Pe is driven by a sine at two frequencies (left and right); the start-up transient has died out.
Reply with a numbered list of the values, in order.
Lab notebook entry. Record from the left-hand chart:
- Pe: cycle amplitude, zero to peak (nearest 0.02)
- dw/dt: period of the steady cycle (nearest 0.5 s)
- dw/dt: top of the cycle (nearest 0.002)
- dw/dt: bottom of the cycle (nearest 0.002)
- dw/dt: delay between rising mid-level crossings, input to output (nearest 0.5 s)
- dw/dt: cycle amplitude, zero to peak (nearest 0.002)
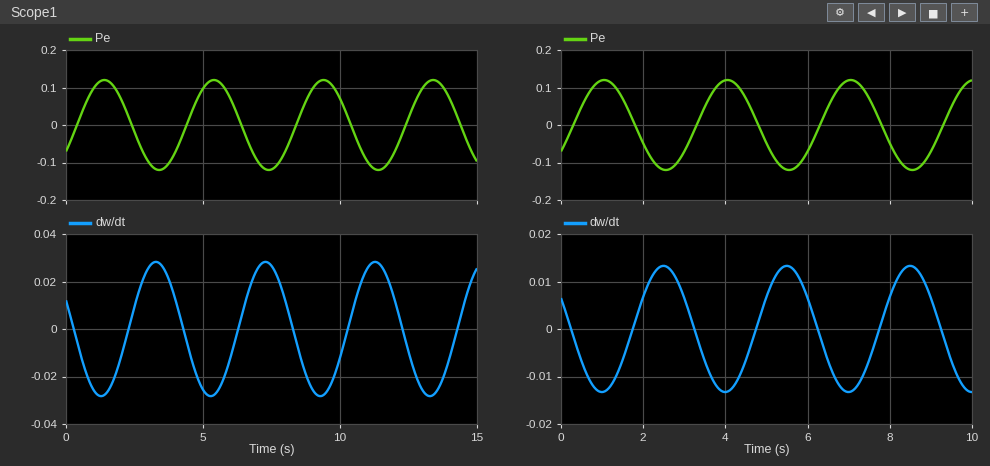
1. 0.12
2. 4.0 s
3. 0.028
4. -0.028
5. 2.0 s
6. 0.028
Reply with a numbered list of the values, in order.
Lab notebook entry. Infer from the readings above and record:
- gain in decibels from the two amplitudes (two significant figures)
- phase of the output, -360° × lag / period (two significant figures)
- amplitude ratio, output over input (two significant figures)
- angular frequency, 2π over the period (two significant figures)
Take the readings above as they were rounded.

1. -13 dB
2. -180°
3. 0.23
4. 1.6 rad/s
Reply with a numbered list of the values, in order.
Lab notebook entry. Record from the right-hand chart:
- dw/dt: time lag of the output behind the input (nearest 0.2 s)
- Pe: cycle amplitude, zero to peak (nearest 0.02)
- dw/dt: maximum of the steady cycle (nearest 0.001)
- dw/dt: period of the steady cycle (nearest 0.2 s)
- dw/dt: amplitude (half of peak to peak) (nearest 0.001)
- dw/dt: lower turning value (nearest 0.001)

1. 1.4 s
2. 0.12
3. 0.013
4. 3.0 s
5. 0.013
6. -0.013
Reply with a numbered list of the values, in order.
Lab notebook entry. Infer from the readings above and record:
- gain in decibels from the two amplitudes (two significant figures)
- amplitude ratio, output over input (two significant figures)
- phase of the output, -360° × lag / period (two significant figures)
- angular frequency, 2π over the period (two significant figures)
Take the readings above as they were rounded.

1. -19 dB
2. 0.11
3. -170°
4. 2.1 rad/s
